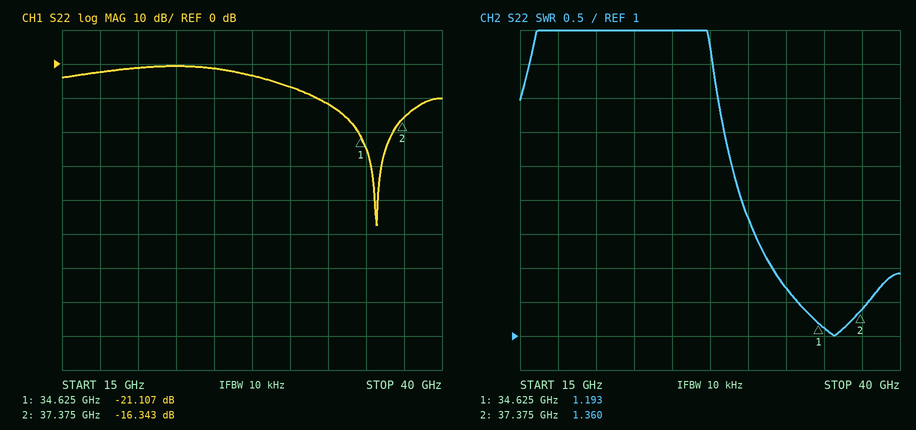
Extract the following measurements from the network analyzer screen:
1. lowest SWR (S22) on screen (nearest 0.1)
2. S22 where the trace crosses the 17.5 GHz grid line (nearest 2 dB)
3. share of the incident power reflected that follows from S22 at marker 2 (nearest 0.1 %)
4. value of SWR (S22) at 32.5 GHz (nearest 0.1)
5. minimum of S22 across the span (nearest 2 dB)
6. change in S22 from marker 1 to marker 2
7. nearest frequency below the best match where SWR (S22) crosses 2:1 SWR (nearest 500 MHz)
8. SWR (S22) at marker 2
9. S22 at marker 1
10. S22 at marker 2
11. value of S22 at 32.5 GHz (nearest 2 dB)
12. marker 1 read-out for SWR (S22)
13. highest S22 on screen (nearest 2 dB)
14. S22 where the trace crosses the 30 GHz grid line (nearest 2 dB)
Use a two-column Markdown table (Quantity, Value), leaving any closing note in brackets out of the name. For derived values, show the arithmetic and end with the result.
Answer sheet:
| Quantity | Value |
|---|---|
| lowest SWR (S22) on screen | 1.0 |
| S22 where the trace crosses the 17.5 GHz grid line | -2 dB |
| share of the incident power reflected that follows from S22 at marker 2 | 10^(-16.343/10) ≈ 2.3 % |
| value of SWR (S22) at 32.5 GHz | 1.7 |
| minimum of S22 across the span | -48 dB |
| change in S22 from marker 1 to marker 2 | -16.343 − (-21.107) = 4.764 dB |
| nearest frequency below the best match where SWR (S22) crosses 2:1 SWR | 31.5 GHz |
| SWR (S22) at marker 2 | 1.360 |
| S22 at marker 1 | -21.107 dB |
| S22 at marker 2 | -16.343 dB |
| value of S22 at 32.5 GHz | -12 dB |
| marker 1 read-out for SWR | 1.193 |
| highest S22 on screen | 0 dB |
| S22 where the trace crosses the 30 GHz grid line | -6 dB |
